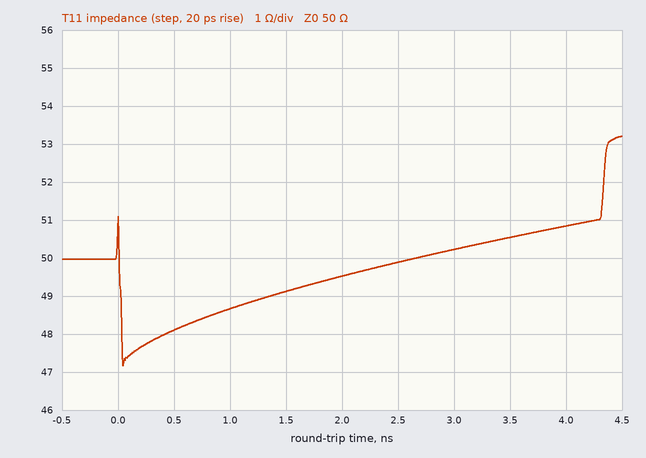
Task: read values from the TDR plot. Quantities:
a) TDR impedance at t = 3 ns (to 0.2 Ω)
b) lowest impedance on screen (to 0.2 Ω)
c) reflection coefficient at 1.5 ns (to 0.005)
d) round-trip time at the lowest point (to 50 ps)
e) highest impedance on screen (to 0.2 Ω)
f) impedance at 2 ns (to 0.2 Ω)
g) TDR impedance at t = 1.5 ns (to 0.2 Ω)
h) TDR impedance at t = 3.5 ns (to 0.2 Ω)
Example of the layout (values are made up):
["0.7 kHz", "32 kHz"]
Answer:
["50.2 Ω", "47.2 Ω", "-0.010", "50 ps", "53.2 Ω", "49.6 Ω", "49.2 Ω", "50.6 Ω"]
